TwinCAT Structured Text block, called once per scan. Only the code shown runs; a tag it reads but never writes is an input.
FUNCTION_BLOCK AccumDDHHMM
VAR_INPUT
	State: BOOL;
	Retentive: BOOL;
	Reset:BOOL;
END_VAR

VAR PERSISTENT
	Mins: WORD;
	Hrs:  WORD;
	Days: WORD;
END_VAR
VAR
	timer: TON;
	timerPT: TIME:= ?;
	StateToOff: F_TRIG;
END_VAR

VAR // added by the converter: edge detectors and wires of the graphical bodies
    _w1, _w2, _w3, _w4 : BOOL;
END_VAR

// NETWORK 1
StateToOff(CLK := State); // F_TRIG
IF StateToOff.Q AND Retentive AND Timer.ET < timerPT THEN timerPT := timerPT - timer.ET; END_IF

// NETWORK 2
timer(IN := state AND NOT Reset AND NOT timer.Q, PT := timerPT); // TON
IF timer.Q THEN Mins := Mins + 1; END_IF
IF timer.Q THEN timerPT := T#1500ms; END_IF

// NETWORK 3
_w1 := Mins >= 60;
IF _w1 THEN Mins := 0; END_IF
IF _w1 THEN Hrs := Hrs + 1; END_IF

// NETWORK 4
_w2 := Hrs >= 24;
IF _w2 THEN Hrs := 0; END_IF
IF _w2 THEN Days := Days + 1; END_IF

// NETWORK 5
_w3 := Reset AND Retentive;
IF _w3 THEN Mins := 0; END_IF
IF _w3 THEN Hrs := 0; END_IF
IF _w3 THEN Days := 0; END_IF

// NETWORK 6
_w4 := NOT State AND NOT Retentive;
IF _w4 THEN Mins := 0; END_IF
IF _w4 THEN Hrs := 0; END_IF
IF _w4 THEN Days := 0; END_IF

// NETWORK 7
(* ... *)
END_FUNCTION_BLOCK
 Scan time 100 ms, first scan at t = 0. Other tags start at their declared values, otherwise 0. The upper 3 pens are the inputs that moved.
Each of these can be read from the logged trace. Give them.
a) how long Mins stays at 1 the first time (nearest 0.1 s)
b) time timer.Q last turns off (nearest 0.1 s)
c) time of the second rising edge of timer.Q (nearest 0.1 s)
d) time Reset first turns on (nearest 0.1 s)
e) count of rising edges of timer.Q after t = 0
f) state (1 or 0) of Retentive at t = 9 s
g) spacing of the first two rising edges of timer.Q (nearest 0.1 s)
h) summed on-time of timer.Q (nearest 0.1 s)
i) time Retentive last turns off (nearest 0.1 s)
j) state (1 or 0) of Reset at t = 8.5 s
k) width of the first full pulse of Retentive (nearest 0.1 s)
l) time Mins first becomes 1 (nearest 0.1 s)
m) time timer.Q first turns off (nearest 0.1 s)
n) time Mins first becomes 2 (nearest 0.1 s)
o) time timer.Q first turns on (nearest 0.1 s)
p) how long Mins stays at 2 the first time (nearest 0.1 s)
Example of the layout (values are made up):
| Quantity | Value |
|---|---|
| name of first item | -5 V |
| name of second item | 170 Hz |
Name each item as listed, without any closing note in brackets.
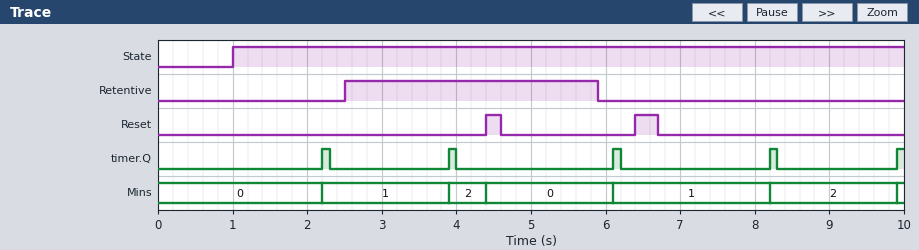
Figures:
| Quantity | Value |
|---|---|
| how long Mins stays at 1 the first time | 1.7 s |
| time timer.Q last turns off | 8.3 s |
| time of the second rising edge of timer.Q | 3.9 s |
| time Reset first turns on | 4.4 s |
| count of rising edges of timer.Q after t = 0 | 5 |
| state (1 or 0) of Retentive at t = 9 s | 0 |
| spacing of the first two rising edges of timer.Q | 1.7 s |
| summed on-time of timer.Q | 0.5 s |
| time Retentive last turns off | 5.9 s |
| state (1 or 0) of Reset at t = 8.5 s | 0 |
| width of the first full pulse of Retentive | 3.4 s |
| time Mins first becomes 1 | 2.2 s |
| time timer.Q first turns off | 2.3 s |
| time Mins first becomes 2 | 3.9 s |
| time timer.Q first turns on | 2.2 s |
| how long Mins stays at 2 the first time | 0.5 s |
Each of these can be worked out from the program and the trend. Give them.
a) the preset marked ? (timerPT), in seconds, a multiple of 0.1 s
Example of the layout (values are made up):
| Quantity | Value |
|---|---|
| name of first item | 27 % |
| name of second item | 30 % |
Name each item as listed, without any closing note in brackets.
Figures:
| Quantity | Value |
|---|---|
| the preset marked ? (timerPT), in seconds, a multiple of 0.1 s | 1.2 s |
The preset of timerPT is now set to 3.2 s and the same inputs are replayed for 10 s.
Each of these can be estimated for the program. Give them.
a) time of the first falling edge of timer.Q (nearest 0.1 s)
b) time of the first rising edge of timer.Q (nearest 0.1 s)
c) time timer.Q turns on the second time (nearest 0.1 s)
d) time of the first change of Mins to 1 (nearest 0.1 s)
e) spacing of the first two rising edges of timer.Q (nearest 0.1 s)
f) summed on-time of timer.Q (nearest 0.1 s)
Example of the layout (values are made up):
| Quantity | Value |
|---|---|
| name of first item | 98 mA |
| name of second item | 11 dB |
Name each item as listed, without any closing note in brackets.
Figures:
| Quantity | Value |
|---|---|
| time of the first falling edge of timer.Q | 4.3 s |
| time of the first rising edge of timer.Q | 4.2 s |
| time timer.Q turns on the second time | 6.1 s |
| time of the first change of Mins to 1 | 4.2 s |
| spacing of the first two rising edges of timer.Q | 1.9 s |
| summed on-time of timer.Q | 0.4 s |
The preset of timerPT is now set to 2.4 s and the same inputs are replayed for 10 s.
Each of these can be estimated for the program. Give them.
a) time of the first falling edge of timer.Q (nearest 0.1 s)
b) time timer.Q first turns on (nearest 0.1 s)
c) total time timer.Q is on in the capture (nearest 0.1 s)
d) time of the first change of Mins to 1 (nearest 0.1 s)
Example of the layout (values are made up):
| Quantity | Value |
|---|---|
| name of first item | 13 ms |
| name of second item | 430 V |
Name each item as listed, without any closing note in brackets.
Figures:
| Quantity | Value |
|---|---|
| time of the first falling edge of timer.Q | 3.5 s |
| time timer.Q first turns on | 3.4 s |
| total time timer.Q is on in the capture | 0.4 s |
| time of the first change of Mins to 1 | 3.4 s |
